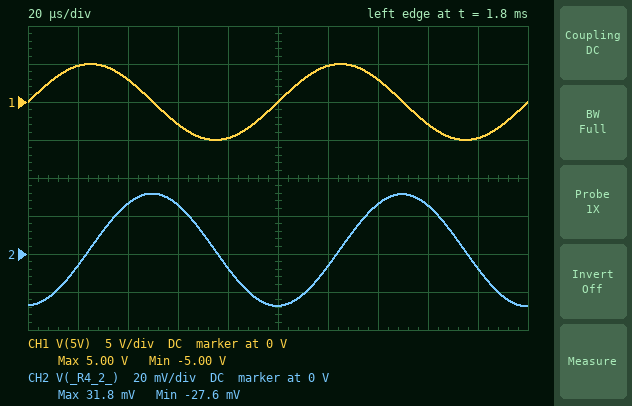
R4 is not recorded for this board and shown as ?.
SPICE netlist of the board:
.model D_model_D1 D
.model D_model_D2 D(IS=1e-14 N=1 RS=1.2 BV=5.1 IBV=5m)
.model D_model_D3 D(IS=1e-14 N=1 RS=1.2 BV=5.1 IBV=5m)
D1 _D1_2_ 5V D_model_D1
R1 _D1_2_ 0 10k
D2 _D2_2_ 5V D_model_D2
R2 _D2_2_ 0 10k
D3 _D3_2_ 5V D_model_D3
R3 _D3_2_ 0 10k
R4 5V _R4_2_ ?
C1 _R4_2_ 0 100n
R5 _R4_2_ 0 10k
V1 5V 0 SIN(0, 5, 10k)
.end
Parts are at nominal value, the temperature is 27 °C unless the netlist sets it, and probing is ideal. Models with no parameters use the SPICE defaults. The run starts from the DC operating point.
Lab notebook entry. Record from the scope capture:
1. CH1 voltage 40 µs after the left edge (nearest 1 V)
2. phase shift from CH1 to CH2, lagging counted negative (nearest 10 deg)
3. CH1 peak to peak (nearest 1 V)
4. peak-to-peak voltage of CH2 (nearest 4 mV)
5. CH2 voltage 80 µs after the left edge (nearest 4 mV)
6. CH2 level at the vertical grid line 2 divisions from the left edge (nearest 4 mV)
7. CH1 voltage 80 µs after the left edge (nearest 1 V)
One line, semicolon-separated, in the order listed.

3 V; -90 deg; 10 V; 60 mV; -8 mV; 28 mV; -5 V
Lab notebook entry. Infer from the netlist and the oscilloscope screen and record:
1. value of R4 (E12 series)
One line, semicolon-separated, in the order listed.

27 kΩ
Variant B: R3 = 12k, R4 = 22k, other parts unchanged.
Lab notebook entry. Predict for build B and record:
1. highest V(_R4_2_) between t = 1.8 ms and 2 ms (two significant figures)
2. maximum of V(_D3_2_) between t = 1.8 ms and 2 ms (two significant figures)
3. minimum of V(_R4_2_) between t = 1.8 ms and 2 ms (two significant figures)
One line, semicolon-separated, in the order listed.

39 mV; 73 mV; -34 mV
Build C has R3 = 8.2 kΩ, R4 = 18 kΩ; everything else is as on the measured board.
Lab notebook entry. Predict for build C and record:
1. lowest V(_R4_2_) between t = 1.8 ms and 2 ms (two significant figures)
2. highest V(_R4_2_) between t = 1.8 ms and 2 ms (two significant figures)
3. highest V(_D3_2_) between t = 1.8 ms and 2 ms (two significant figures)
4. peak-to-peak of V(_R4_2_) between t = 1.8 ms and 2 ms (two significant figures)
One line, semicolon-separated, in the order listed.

-42 mV; 47 mV; 66 mV; 89 mV
